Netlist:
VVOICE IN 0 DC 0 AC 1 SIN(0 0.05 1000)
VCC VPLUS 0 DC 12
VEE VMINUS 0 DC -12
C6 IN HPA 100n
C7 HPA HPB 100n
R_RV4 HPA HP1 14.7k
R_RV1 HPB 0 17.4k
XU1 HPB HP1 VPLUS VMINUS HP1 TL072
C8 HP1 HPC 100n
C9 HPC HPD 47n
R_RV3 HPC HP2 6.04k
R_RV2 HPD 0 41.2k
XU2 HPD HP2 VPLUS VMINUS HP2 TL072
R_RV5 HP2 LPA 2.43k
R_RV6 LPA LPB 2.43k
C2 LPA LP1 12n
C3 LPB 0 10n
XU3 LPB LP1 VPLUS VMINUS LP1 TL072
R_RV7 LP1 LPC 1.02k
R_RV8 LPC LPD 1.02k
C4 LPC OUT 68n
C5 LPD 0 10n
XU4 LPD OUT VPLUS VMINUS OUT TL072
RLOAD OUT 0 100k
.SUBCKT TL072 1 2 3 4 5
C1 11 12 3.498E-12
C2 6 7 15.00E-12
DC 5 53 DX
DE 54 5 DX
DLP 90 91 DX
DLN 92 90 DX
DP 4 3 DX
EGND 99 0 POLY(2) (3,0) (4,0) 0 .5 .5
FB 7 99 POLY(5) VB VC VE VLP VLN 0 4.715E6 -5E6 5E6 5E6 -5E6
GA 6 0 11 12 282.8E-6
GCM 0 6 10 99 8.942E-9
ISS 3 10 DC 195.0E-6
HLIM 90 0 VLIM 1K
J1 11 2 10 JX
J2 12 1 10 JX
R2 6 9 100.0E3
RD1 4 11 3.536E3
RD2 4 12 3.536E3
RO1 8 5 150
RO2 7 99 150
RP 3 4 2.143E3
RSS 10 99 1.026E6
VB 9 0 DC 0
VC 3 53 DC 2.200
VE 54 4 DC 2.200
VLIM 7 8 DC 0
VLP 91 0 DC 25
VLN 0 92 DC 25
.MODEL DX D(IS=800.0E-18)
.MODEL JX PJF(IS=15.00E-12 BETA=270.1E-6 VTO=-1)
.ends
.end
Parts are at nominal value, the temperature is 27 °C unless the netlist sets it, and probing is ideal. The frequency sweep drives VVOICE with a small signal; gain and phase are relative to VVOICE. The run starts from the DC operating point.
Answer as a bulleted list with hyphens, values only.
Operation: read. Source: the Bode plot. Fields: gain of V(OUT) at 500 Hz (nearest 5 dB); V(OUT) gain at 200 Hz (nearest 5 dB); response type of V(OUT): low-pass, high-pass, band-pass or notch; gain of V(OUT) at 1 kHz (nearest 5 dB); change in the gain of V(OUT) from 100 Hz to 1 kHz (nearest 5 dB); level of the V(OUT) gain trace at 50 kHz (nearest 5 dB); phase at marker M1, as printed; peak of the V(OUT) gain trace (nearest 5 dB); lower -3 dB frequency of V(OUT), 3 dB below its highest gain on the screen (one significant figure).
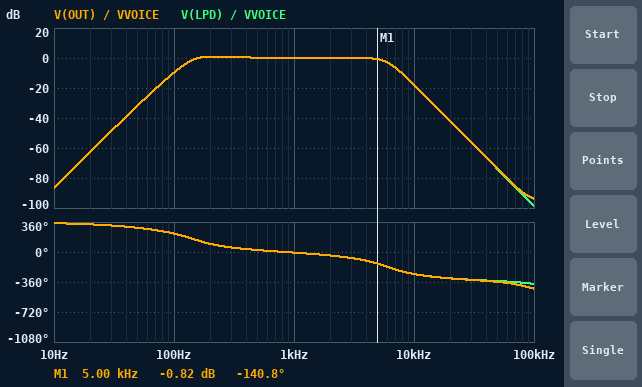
- 0 dB
- 0 dB
- band-pass
- 0 dB
- 10 dB
- -75 dB
- -140.8 deg
- 0 dB
- 100 Hz
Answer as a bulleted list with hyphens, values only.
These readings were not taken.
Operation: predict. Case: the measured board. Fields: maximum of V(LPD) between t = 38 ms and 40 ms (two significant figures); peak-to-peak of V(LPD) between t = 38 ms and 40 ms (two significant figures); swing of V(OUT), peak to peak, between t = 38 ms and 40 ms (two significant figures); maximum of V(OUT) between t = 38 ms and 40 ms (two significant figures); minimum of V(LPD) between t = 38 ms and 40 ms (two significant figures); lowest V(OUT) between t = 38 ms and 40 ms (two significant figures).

- 50 mV
- 100 mV
- 100 mV
- 50 mV
- -50 mV
- -50 mV
